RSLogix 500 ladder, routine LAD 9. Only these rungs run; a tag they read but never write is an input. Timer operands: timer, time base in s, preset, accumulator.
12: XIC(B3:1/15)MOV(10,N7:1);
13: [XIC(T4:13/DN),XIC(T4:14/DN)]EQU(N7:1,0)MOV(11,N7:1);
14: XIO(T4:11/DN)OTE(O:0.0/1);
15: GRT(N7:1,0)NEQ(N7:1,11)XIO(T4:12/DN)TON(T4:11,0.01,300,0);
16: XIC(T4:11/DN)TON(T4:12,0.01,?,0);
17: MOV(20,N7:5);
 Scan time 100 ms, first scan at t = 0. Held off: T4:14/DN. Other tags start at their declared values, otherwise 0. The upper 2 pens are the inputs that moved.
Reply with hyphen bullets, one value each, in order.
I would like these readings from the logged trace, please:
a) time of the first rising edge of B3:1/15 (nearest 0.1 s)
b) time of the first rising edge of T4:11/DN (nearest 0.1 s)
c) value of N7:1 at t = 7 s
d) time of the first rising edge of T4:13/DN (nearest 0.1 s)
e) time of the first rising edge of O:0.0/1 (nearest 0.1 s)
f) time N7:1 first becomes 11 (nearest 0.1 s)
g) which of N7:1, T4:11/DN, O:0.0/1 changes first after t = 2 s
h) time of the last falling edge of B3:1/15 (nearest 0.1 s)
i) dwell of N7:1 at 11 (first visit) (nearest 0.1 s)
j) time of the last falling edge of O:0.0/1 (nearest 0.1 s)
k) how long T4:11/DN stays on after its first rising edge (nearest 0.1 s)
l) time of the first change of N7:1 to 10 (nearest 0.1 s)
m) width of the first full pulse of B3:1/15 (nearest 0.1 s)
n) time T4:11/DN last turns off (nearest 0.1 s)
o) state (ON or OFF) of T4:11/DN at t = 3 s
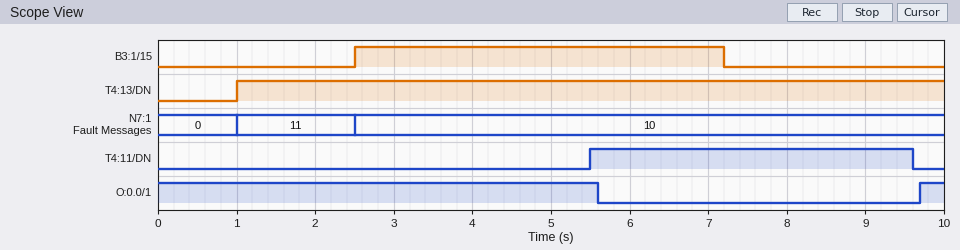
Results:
- 2.5 s
- 5.5 s
- 10
- 1.0 s
- 9.7 s
- 1.0 s
- N7:1
- 7.2 s
- 1.5 s
- 5.6 s
- 4.1 s
- 2.5 s
- 4.7 s
- 9.6 s
- OFF
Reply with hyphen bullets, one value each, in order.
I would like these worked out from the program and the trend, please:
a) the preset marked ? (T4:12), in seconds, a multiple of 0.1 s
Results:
- 4.0 s
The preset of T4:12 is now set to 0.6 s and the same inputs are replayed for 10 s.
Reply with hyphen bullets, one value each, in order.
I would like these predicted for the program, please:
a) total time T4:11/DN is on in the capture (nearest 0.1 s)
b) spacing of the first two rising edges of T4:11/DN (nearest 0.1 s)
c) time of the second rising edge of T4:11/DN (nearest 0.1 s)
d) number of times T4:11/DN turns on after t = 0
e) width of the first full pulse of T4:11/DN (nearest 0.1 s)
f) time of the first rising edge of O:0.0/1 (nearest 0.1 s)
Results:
- 1.4 s
- 3.8 s
- 9.3 s
- 2
- 0.7 s
- 6.3 s
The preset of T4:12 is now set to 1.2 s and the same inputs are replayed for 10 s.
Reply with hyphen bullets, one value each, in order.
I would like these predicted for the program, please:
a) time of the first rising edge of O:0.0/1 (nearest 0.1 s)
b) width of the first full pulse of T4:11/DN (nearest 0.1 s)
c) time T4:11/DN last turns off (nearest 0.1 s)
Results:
- 6.9 s
- 1.3 s
- 6.8 s
